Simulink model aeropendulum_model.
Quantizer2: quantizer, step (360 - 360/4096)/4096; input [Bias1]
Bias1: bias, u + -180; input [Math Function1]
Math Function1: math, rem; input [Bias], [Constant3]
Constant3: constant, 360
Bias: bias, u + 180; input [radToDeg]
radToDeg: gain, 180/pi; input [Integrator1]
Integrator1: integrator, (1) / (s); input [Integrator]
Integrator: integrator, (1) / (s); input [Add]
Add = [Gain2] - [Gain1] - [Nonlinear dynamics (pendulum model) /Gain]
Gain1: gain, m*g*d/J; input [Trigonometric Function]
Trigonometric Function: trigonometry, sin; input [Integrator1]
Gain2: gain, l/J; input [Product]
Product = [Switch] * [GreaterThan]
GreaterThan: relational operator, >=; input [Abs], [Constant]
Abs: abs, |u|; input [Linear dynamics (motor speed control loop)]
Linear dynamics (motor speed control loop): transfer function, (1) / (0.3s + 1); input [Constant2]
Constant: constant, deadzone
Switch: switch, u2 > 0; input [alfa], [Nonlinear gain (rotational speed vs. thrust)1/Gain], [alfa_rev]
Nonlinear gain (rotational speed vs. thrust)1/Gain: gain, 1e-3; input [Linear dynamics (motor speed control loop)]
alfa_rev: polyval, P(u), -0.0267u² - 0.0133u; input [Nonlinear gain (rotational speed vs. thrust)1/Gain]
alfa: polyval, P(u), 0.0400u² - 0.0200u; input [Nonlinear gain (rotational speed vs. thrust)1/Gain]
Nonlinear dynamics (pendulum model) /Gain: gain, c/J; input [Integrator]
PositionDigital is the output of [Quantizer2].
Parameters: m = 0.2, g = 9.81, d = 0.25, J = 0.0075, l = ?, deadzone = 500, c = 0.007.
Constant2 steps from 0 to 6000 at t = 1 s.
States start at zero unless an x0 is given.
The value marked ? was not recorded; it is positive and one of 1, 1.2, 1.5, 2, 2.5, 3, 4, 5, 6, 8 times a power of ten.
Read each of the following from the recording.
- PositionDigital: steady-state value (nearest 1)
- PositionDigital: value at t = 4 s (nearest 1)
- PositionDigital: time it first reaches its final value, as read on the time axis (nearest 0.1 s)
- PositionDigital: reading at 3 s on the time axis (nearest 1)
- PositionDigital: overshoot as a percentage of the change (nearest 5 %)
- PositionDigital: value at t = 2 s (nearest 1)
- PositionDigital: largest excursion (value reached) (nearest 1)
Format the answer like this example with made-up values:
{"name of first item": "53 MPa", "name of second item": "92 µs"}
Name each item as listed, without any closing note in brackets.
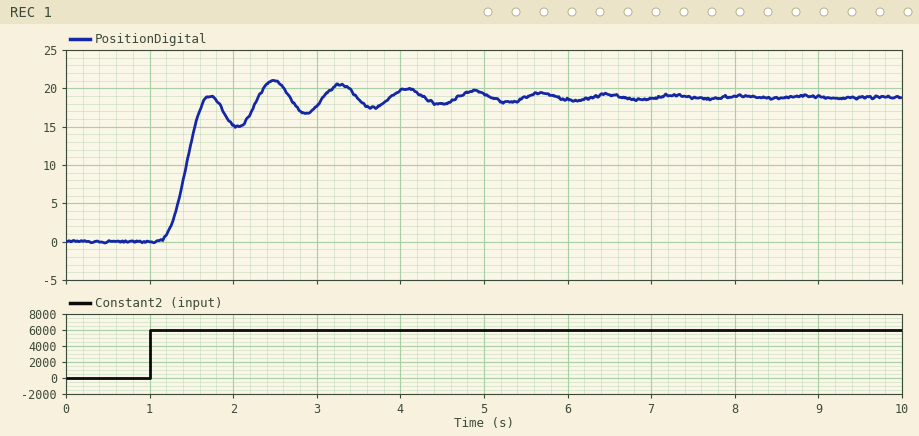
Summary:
{"PositionDigital: steady-state value": "19", "PositionDigital: value at t = 4 s": "20", "PositionDigital: time it first reaches its final value, as read on the time axis": "1.7 s", "PositionDigital: reading at 3 s on the time axis": "18", "PositionDigital: overshoot as a percentage of the change": "10 %", "PositionDigital: value at t = 2 s": "15", "PositionDigital: largest excursion (value reached)": "21"}
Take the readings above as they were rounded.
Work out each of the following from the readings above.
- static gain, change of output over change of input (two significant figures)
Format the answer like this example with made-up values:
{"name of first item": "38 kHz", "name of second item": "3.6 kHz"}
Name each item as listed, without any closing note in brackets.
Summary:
{"static gain, change of output over change of input": "0.0032"}
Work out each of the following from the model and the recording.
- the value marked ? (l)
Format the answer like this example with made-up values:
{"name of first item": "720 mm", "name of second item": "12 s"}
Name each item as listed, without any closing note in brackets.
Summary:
{"the value marked ?": "0.12"}
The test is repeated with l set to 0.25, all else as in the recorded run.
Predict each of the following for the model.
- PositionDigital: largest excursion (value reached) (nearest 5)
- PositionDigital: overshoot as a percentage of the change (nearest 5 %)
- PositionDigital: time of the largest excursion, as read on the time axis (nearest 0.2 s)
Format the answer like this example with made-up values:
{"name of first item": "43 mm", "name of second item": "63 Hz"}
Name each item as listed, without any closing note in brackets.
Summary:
{"PositionDigital: largest excursion (value reached)": "45", "PositionDigital: overshoot as a percentage of the change": "10 %", "PositionDigital: time of the largest excursion, as read on the time axis": "2.6 s"}
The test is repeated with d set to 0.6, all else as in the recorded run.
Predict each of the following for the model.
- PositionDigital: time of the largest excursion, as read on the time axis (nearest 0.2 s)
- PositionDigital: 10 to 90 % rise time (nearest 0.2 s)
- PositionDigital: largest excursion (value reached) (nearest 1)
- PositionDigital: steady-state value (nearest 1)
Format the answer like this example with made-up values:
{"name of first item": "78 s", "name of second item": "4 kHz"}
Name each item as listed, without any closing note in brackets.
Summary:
{"PositionDigital: time of the largest excursion, as read on the time axis": "2.4 s", "PositionDigital: 10 to 90 % rise time": "0.6 s", "PositionDigital: largest excursion (value reached)": "8", "PositionDigital: steady-state value": "8"}
